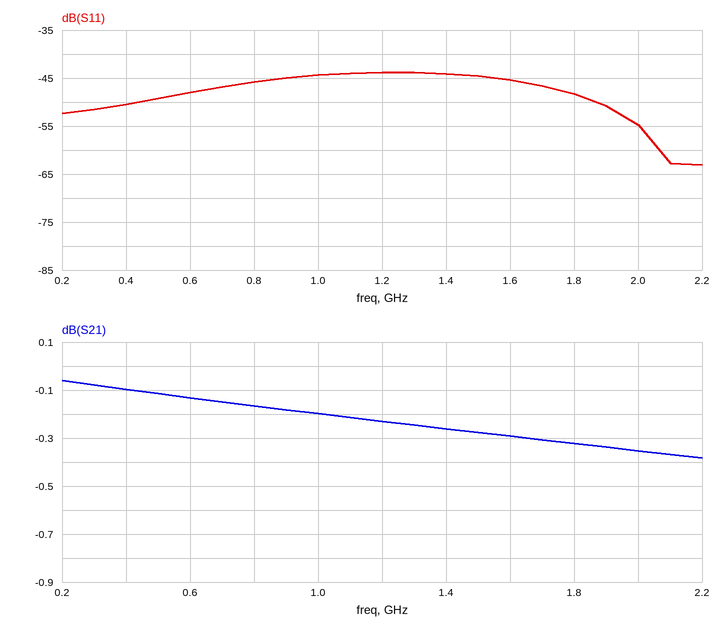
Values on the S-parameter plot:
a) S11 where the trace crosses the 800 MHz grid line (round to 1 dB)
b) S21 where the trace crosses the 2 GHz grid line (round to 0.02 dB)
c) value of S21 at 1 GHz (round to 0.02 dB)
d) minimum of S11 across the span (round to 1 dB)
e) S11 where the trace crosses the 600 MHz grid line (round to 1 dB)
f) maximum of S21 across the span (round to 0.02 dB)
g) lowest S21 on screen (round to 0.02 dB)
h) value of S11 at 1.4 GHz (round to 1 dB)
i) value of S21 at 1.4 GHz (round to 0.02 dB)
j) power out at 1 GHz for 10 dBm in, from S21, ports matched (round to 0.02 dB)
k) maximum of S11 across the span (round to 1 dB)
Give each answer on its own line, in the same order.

-46 dB
-0.36 dB
-0.20 dB
-63 dB
-48 dB
-0.06 dB
-0.38 dB
-44 dB
-0.26 dB
9.80 dBm
-44 dB
